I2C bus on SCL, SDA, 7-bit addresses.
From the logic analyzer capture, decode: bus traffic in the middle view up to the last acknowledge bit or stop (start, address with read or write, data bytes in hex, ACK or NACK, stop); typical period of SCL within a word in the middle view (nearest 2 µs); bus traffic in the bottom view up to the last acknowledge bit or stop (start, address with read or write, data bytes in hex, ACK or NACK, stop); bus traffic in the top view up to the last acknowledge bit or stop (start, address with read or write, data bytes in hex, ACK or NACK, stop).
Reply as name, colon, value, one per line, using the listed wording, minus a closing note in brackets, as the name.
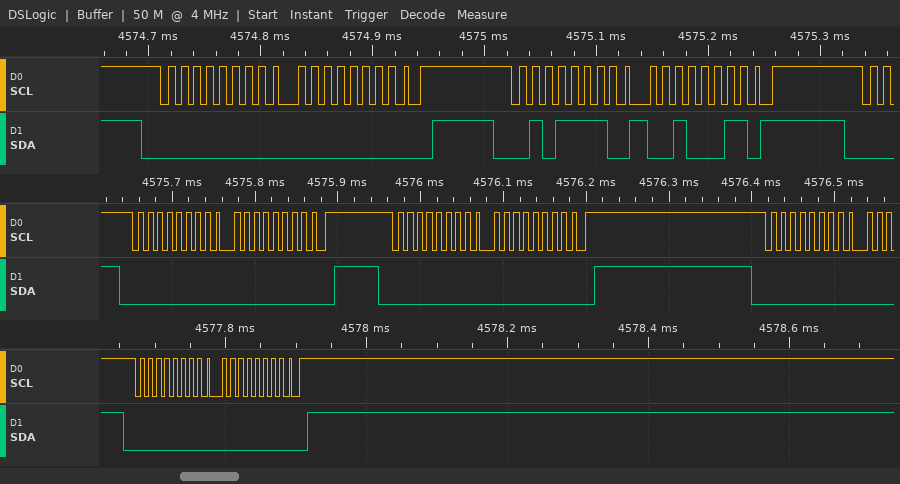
bus traffic in the middle view up to the last acknowledge bit or stop: start, address 00 write ACK, 00 ACK, stop, start, address 00 write ACK, 00 ACK, stop, start, address 00 write ACK
typical period of SCL within a word in the middle view: 12 µs
bus traffic in the bottom view up to the last acknowledge bit or stop: start, address 00 write ACK, 00 ACK, stop
bus traffic in the top view up to the last acknowledge bit or stop: start, address 00 write ACK, 00 ACK, stop, start, address 2F write ACK, 23 ACK
